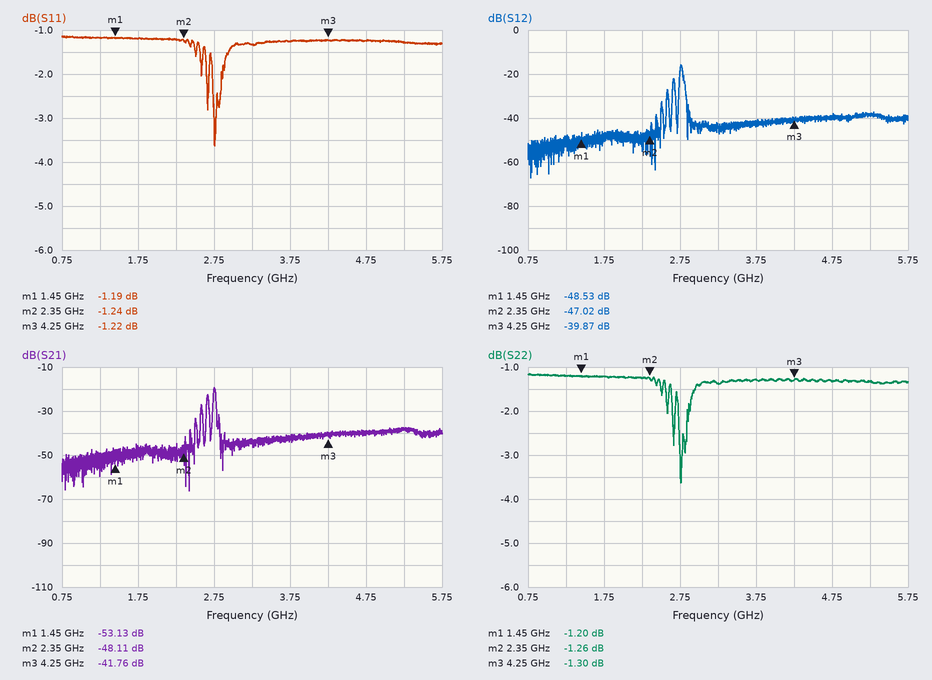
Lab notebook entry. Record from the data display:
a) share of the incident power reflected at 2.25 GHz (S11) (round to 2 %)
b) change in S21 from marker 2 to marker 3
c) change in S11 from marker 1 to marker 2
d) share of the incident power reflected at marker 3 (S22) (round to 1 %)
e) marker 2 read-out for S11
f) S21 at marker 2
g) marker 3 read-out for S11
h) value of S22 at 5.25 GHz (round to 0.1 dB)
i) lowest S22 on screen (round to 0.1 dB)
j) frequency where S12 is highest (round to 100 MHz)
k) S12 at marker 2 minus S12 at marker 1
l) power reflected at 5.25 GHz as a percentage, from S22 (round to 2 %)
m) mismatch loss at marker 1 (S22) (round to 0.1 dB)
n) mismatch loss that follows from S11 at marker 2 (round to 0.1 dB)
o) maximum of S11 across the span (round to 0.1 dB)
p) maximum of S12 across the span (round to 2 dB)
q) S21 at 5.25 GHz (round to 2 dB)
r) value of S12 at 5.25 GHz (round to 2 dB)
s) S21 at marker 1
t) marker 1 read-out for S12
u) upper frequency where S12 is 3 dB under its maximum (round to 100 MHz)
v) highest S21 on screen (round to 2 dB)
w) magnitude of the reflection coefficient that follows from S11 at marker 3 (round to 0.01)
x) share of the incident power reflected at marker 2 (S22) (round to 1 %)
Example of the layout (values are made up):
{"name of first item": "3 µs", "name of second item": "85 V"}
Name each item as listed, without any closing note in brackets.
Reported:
{"share of the incident power reflected at 2.25 GHz (S11)": "76 %", "change in S21 from marker 2 to marker 3": "6.35 dB", "change in S11 from marker 1 to marker 2": "-0.05 dB", "share of the incident power reflected at marker 3 (S22)": "74 %", "marker 2 read-out for S11": "-1.24 dB", "S21 at marker 2": "-48.11 dB", "marker 3 read-out for S11": "-1.22 dB", "value of S22 at 5.25 GHz": "-1.3 dB", "lowest S22 on screen": "-3.6 dB", "frequency where S12 is highest": "2.8 GHz", "S12 at marker 2 minus S12 at marker 1": "1.51 dB", "power reflected at 5.25 GHz as a percentage, from S22": "74 %", "mismatch loss at marker 1 (S22)": "6.2 dB", "mismatch loss that follows from S11 at marker 2": "6.0 dB", "maximum of S11 across the span": "-1.1 dB", "maximum of S12 across the span": "-16 dB", "S21 at 5.25 GHz": "-38 dB", "value of S12 at 5.25 GHz": "-38 dB", "S21 at marker 1": "-53.13 dB", "marker 1 read-out for S12": "-48.53 dB", "upper frequency where S12 is 3 dB under its maximum": "2.8 GHz", "highest S21 on screen": "-20 dB", "magnitude of the reflection coefficient that follows from S11 at marker 3": "0.87", "share of the incident power reflected at marker 2 (S22)": "75 %"}
